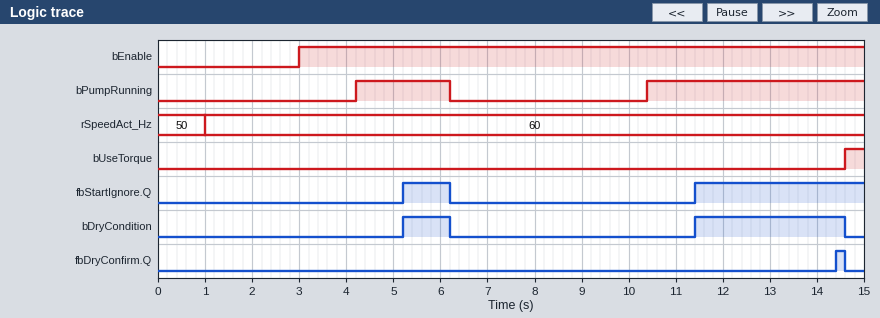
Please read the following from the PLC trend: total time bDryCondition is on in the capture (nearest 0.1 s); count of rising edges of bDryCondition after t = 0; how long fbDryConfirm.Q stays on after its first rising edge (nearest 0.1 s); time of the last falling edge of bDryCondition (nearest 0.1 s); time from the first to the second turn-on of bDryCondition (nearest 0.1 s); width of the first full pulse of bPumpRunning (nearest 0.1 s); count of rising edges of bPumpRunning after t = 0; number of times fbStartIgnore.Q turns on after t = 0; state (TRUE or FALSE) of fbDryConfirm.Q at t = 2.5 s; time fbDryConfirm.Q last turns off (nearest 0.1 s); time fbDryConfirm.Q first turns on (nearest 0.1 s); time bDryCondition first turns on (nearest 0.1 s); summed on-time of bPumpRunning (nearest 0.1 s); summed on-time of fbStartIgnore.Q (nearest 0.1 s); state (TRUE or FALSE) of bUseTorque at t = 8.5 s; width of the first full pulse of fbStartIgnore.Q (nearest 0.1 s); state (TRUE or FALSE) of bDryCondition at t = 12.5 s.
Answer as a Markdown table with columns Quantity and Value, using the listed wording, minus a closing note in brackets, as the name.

| Quantity | Value |
|---|---|
| total time bDryCondition is on in the capture | 4.2 s |
| count of rising edges of bDryCondition after t = 0 | 2 |
| how long fbDryConfirm.Q stays on after its first rising edge | 0.2 s |
| time of the last falling edge of bDryCondition | 14.6 s |
| time from the first to the second turn-on of bDryCondition | 6.2 s |
| width of the first full pulse of bPumpRunning | 2.0 s |
| count of rising edges of bPumpRunning after t = 0 | 2 |
| number of times fbStartIgnore.Q turns on after t = 0 | 2 |
| state (TRUE or FALSE) of fbDryConfirm.Q at t = 2.5 s | FALSE |
| time fbDryConfirm.Q last turns off | 14.6 s |
| time fbDryConfirm.Q first turns on | 14.4 s |
| time bDryCondition first turns on | 5.2 s |
| summed on-time of bPumpRunning | 6.6 s |
| summed on-time of fbStartIgnore.Q | 4.6 s |
| state (TRUE or FALSE) of bUseTorque at t = 8.5 s | FALSE |
| width of the first full pulse of fbStartIgnore.Q | 1.0 s |
| state (TRUE or FALSE) of bDryCondition at t = 12.5 s | TRUE |
